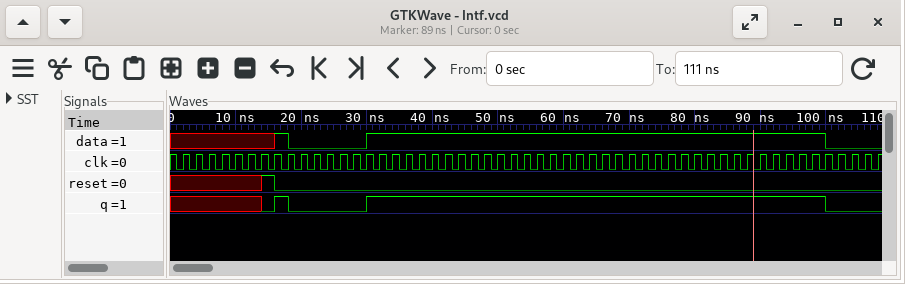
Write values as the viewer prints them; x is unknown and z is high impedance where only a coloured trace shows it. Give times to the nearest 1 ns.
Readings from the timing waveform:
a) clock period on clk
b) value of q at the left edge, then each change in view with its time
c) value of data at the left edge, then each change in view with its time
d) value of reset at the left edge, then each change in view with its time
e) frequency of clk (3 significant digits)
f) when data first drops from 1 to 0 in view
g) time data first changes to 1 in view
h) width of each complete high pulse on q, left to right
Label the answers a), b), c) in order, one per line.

a) 2 ns
b) x, 0 at 14 ns, 1 at 16 ns, 0 at 18 ns, 1 at 30 ns, 0 at 100 ns
c) x, 1 at 16 ns, 0 at 18 ns, 1 at 30 ns, 0 at 100 ns
d) x, 1 at 14 ns, 0 at 16 ns
e) 500 MHz
f) 18 ns
g) 16 ns
h) 2 ns, 70 ns
